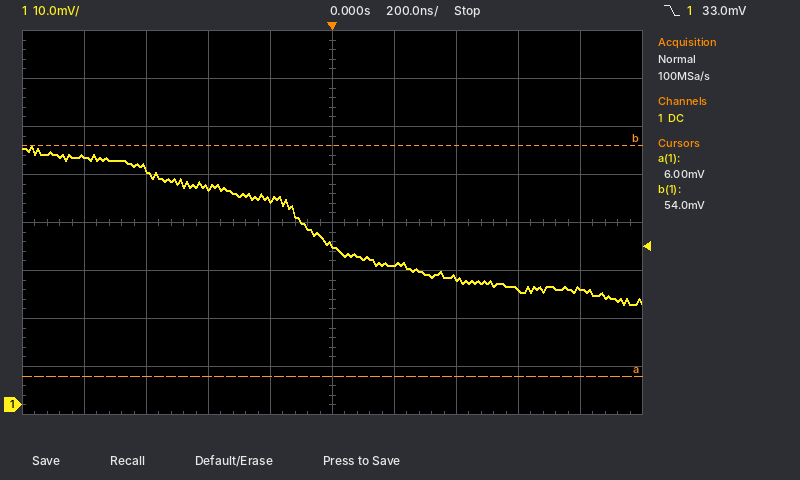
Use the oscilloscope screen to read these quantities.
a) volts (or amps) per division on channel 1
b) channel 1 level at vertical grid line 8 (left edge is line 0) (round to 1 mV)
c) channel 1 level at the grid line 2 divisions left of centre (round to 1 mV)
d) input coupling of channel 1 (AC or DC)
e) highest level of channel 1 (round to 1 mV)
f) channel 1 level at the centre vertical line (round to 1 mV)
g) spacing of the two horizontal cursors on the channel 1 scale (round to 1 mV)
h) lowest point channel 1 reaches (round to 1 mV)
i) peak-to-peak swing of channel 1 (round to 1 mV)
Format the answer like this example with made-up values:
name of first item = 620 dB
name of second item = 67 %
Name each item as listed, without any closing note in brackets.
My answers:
volts (or amps) per division on channel 1 = 10 mV
channel 1 level at vertical grid line 8 (left edge is line 0) = 24 mV
channel 1 level at the grid line 2 divisions left of centre = 45 mV
input coupling of channel 1 = DC
highest level of channel 1 = 54 mV
channel 1 level at the centre vertical line = 33 mV
spacing of the two horizontal cursors on the channel 1 scale = 48 mV
lowest point channel 1 reaches = 21 mV
peak-to-peak swing of channel 1 = 33 mV
